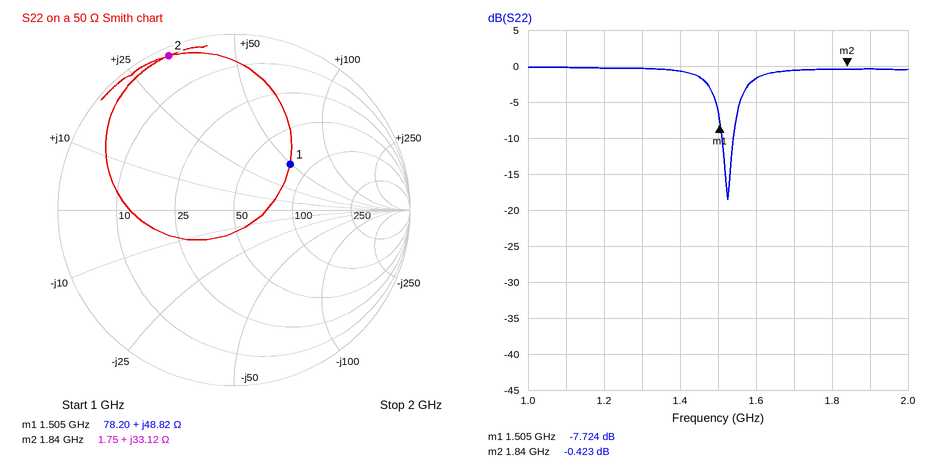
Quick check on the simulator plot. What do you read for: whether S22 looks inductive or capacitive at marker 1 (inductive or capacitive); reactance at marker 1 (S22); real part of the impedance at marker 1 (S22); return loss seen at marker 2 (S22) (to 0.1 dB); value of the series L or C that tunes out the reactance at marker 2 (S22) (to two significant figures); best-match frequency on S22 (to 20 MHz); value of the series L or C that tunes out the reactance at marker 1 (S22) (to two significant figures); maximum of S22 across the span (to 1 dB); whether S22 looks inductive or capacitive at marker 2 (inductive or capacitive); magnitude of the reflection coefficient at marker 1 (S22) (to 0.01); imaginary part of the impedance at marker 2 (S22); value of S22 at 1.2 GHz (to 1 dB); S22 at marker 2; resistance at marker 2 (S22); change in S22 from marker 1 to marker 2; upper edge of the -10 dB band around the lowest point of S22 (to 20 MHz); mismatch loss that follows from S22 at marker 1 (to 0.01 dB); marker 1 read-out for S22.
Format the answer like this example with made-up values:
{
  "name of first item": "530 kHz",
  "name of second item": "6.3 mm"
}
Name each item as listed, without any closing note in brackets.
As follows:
{
  "whether S22 looks inductive or capacitive at marker 1": "inductive",
  "reactance at marker 1": "+48.82 Ω",
  "real part of the impedance at marker 1": "78.20 Ω",
  "return loss seen at marker 2 (S22)": "0.4 dB",
  "value of the series L or C that tunes out the reactance at marker 2 (S22)": "2.6 pF",
  "best-match frequency on S22": "1.52 GHz",
  "value of the series L or C that tunes out the reactance at marker 1 (S22)": "2.2 pF",
  "maximum of S22 across the span": "0 dB",
  "whether S22 looks inductive or capacitive at marker 2": "inductive",
  "magnitude of the reflection coefficient at marker 1 (S22)": "0.41",
  "imaginary part of the impedance at marker 2": "+33.12 Ω",
  "value of S22 at 1.2 GHz": "0 dB",
  "S22 at marker 2": "-0.423 dB",
  "resistance at marker 2": "1.75 Ω",
  "change in S22 from marker 1 to marker 2": "7.301 dB",
  "upper edge of the -10 dB band around the lowest point of S22": "1.54 GHz",
  "mismatch loss that follows from S22 at marker 1": "0.80 dB",
  "marker 1 read-out for S22": "-7.724 dB"
}
